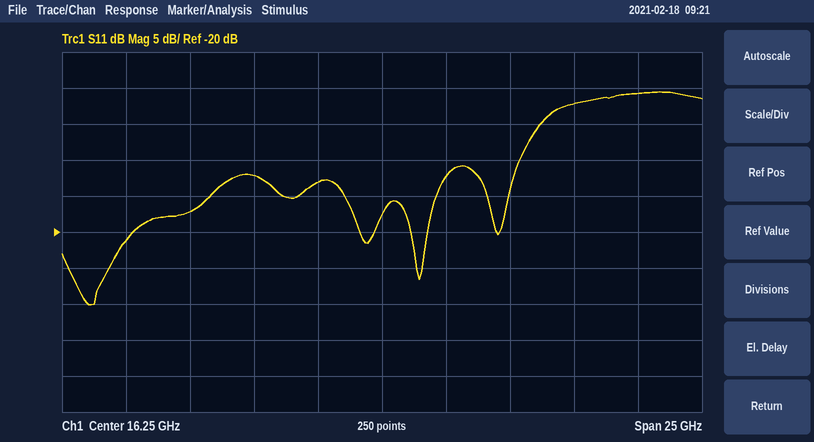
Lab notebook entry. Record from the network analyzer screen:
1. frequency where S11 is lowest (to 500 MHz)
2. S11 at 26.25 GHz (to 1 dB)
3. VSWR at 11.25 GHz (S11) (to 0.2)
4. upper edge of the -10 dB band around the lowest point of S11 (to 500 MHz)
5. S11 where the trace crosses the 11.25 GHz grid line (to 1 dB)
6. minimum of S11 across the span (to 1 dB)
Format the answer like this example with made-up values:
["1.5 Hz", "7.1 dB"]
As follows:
["5.0 GHz", "-1 dB", "1.6", "21.5 GHz", "-12 dB", "-30 dB"]
